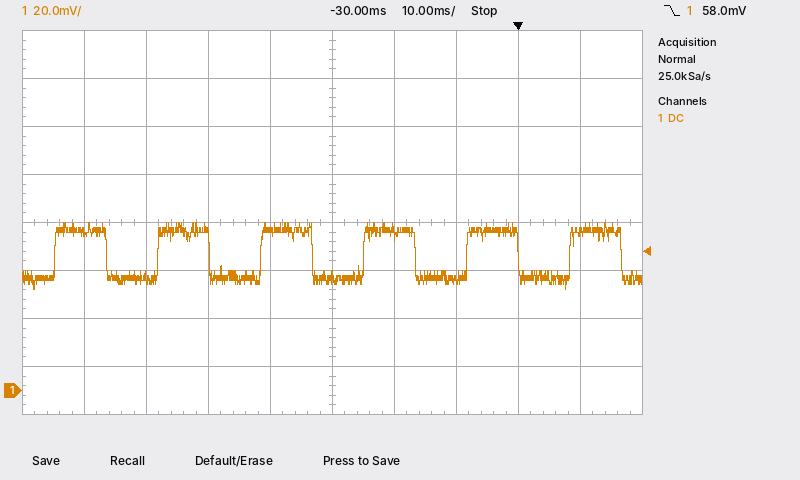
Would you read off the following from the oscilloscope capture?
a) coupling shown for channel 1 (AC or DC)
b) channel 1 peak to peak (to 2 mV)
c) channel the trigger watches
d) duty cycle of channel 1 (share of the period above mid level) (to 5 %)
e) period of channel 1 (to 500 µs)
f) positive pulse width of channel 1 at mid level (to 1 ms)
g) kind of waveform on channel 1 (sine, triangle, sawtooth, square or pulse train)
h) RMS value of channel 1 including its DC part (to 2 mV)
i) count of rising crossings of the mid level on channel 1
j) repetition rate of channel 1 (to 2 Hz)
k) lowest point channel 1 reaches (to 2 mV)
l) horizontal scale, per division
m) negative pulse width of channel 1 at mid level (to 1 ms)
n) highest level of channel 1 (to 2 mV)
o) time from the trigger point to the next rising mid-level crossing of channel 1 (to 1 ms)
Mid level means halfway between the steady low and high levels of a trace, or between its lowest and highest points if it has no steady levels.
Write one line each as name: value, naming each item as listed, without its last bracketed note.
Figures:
coupling shown for channel 1: DC
channel 1 peak to peak: 28 mV
channel the trigger watches: channel 1
duty cycle of channel 1 (share of the period above mid level): 50 %
period of channel 1: 16.5 ms
positive pulse width of channel 1 at mid level: 8 ms
kind of waveform on channel 1: square
RMS value of channel 1 including its DC part: 58 mV
count of rising crossings of the mid level on channel 1: 6
repetition rate of channel 1: 60 Hz
lowest point channel 1 reaches: 42 mV
horizontal scale, per division: 10 ms
negative pulse width of channel 1 at mid level: 8 ms
highest level of channel 1: 70 mV
time from the trigger point to the next rising mid-level crossing of channel 1: 8 ms
